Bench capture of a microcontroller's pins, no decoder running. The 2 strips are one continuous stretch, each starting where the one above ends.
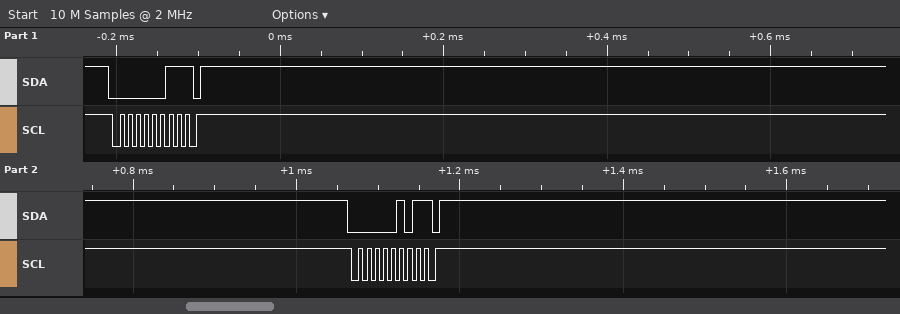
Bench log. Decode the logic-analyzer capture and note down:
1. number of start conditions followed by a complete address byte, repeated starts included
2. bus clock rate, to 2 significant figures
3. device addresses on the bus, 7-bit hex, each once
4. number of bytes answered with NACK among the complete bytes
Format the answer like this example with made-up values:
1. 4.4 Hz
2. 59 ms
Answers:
1. 2
2. 100 kHz
3. 0x01 0x02
4. 2
